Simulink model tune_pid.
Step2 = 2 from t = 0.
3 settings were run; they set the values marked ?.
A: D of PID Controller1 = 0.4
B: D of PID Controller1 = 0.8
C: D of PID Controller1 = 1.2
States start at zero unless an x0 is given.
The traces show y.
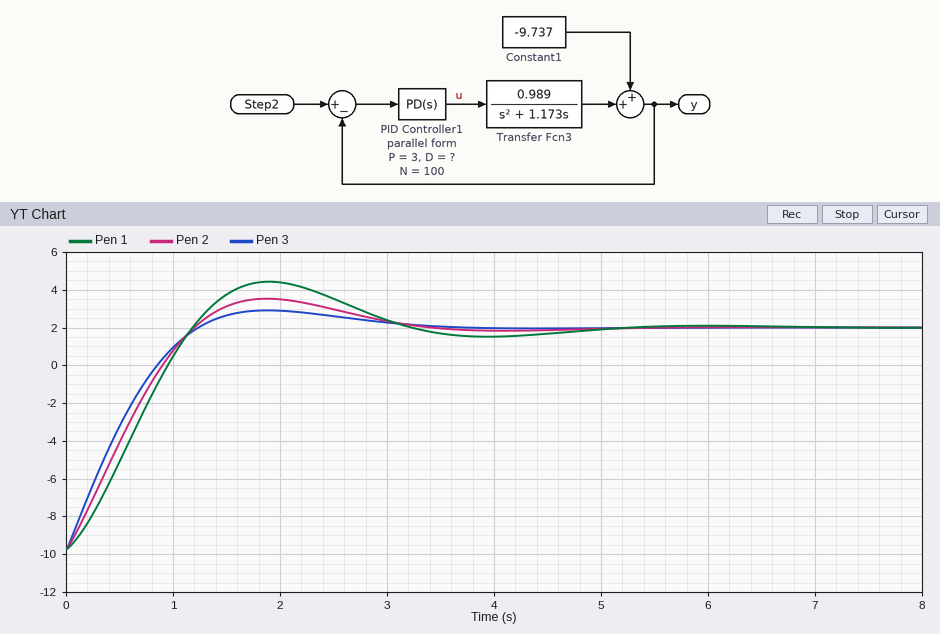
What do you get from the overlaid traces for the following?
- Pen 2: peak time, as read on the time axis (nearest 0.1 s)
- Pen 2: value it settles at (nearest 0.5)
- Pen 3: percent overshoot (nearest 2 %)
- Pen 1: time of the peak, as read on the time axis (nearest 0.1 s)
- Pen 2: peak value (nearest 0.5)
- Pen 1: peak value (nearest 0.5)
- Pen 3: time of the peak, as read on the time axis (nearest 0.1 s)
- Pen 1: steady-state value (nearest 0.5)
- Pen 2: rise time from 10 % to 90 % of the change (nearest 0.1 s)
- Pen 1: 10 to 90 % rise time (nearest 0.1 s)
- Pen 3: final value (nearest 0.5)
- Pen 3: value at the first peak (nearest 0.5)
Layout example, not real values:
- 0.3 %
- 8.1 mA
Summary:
- 1.9 s
- 2.0
- 8 %
- 1.9 s
- 3.5
- 4.5
- 1.9 s
- 2.0
- 0.9 s
- 0.9 s
- 2.0
- 3.0
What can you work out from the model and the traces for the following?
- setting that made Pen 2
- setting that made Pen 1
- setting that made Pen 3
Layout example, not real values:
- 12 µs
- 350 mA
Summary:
- B
- A
- C
